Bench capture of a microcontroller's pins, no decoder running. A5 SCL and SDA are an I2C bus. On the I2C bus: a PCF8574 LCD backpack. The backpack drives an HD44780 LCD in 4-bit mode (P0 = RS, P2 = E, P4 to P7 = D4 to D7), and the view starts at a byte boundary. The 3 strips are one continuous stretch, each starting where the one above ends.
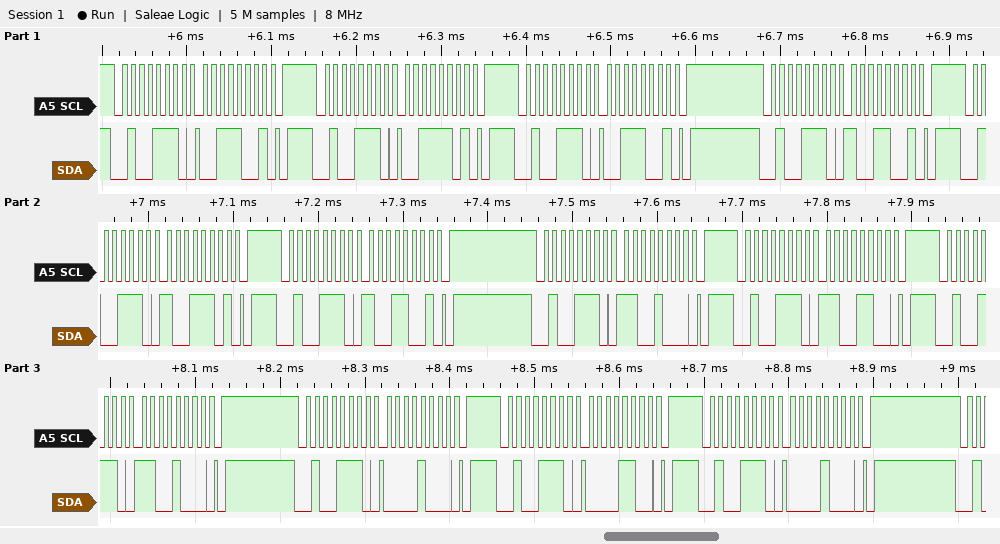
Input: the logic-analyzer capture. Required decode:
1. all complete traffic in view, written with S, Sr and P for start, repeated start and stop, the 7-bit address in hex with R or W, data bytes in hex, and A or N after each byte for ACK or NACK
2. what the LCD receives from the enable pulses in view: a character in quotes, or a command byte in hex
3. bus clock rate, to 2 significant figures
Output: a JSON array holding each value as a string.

["S 27W A 39 A P S 27W A 3D A P S 27W A 39 A P S 27W A 99 A P S 27W A 9D A P S 27W A 99 A P S 27W A C8 A P S 27W A CC A P S 27W A C8 A P S 27W A 08 A P S 27W A 0C A P S 27W A 08 A P", "'9' 0xC0", "100 kHz"]
